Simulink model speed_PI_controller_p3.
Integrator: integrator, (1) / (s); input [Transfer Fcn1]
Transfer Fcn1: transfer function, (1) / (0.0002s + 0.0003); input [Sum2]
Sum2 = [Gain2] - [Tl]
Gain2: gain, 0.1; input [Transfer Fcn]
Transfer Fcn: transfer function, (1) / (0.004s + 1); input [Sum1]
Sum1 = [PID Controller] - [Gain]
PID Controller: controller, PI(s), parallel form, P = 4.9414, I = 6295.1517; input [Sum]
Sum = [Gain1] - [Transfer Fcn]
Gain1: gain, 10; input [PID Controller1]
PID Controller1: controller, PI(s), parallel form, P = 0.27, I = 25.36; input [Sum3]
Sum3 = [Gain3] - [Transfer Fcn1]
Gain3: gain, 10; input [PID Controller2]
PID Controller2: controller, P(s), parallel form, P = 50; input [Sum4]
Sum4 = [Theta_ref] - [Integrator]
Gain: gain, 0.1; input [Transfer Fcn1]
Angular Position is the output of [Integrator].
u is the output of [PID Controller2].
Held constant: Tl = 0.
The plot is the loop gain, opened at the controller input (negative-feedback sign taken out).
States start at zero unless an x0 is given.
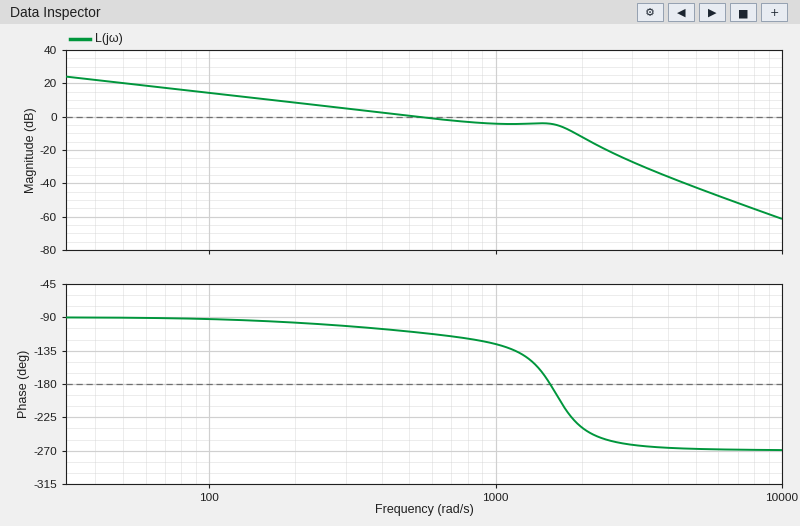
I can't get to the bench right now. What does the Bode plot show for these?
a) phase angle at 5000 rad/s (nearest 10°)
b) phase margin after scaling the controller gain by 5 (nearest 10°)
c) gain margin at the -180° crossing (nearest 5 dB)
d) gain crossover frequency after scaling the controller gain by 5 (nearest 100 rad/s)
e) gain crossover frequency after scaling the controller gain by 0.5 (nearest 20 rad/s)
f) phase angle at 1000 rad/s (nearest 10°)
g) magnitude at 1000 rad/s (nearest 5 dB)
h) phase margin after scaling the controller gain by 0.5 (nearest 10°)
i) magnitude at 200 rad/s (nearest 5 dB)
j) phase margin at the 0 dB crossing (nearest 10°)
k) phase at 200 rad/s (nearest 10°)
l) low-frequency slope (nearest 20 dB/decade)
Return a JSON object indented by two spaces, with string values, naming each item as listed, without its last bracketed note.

{
  "phase angle at 5000 rad/s": "-270°",
  "phase margin after scaling the controller gain by 5": "-60°",
  "gain margin at the -180° crossing": "5 dB",
  "gain crossover frequency after scaling the controller gain by 5": "2100 rad/s",
  "gain crossover frequency after scaling the controller gain by 0.5": "260 rad/s",
  "phase angle at 1000 rad/s": "-130°",
  "magnitude at 1000 rad/s": "-5 dB",
  "phase margin after scaling the controller gain by 0.5": "80°",
  "magnitude at 200 rad/s": "10 dB",
  "phase margin at the 0 dB crossing": "70°",
  "phase at 200 rad/s": "-100°",
  "low-frequency slope": "-20 dB/decade"
}
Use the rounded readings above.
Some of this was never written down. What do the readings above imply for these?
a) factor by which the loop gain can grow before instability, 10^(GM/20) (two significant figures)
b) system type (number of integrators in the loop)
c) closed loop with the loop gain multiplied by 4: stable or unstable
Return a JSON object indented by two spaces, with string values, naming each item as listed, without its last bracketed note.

{
  "factor by which the loop gain can grow before instability, 10^(GM/20)": "1.8",
  "system type": "1",
  "closed loop with the loop gain multiplied by 4: stable or unstable": "unstable"
}
